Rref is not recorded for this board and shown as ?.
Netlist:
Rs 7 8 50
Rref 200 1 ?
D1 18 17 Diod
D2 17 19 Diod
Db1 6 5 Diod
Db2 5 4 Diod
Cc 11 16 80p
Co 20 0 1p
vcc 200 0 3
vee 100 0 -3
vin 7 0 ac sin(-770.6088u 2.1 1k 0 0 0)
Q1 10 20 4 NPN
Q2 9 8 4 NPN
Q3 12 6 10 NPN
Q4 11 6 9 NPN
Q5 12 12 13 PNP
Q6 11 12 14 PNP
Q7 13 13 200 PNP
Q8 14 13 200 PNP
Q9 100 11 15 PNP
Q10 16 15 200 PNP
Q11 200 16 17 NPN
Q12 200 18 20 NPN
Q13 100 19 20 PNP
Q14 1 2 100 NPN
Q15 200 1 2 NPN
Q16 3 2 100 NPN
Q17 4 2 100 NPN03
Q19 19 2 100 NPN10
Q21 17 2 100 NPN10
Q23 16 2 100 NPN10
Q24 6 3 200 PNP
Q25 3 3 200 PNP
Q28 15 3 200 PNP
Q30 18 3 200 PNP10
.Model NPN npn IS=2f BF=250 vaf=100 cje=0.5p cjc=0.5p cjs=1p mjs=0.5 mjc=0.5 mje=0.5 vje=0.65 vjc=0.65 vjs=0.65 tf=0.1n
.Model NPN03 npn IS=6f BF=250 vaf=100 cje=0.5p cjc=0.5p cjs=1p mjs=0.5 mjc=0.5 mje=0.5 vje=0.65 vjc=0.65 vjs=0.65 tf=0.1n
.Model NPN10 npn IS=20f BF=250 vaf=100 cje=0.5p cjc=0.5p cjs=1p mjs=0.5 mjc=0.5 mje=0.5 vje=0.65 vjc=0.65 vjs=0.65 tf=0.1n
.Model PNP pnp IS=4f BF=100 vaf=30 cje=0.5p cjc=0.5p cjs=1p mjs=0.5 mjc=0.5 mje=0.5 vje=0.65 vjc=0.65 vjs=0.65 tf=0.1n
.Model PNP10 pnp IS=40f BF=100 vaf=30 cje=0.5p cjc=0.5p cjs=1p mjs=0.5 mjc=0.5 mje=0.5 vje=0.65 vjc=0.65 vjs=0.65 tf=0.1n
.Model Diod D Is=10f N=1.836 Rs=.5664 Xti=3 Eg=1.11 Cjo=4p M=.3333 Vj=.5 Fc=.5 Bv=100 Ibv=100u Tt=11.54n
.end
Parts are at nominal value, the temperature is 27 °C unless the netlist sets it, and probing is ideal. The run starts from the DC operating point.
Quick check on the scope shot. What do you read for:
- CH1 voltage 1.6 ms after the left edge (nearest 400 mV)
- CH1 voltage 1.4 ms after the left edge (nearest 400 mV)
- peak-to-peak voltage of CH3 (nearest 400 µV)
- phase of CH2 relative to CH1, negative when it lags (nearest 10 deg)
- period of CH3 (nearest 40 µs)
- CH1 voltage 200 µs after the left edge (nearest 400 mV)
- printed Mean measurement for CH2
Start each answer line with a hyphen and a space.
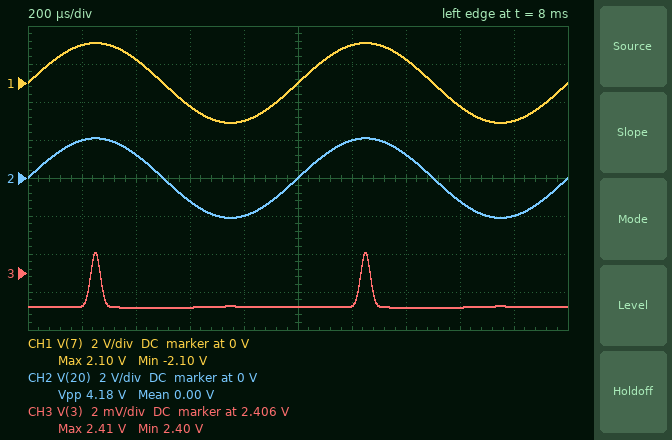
- -1.2 V
- 1.2 V
- 2.8 mV
- 0 deg
- 1.00 ms
- 2.0 V
- 0.00 V
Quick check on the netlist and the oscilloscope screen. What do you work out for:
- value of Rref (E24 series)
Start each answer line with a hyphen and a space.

- 110 kΩ
